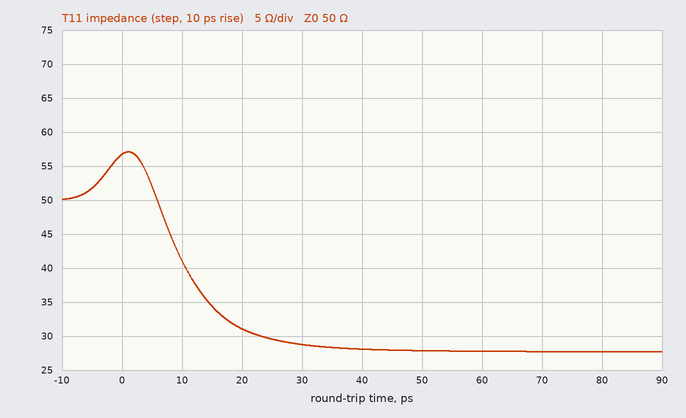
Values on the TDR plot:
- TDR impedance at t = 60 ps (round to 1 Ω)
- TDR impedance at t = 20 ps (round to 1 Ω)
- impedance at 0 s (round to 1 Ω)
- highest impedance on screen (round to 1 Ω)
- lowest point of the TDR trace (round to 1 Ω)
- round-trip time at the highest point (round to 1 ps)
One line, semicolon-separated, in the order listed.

28 Ω; 31 Ω; 57 Ω; 57 Ω; 28 Ω; 1 ps
